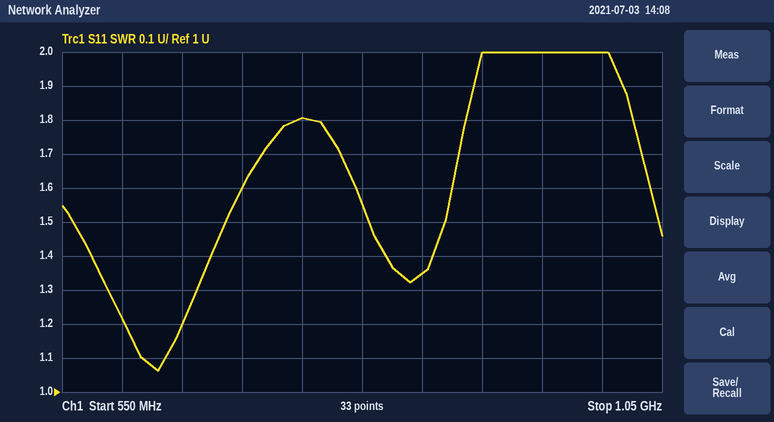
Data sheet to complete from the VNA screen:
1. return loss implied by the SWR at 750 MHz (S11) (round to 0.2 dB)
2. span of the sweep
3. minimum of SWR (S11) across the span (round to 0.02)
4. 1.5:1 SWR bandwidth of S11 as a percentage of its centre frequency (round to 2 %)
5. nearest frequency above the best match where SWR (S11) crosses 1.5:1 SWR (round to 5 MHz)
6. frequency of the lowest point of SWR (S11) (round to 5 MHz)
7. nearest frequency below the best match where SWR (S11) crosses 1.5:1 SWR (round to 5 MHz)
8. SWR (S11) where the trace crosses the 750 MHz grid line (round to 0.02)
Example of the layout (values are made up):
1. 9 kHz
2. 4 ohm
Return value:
1. 10.8 dB
2. 500 MHz
3. 1.06
4. 20 %
5. 685 MHz
6. 630 MHz
7. 560 MHz
8. 1.80
